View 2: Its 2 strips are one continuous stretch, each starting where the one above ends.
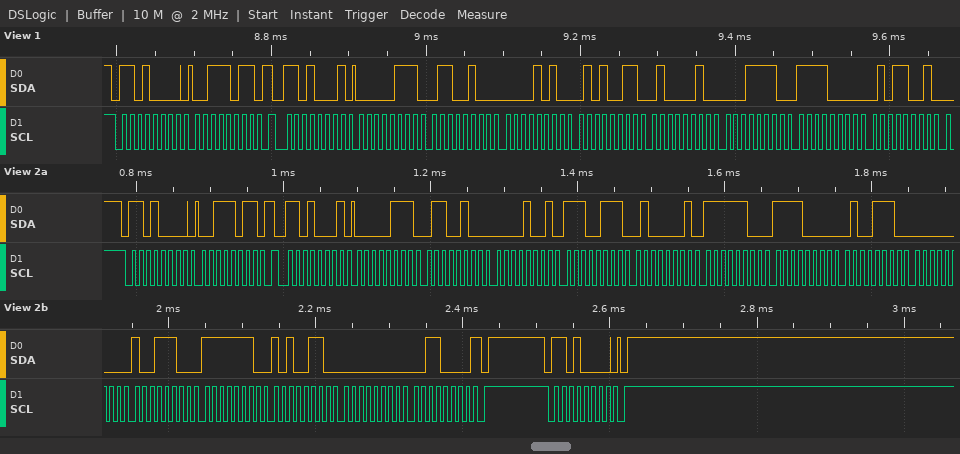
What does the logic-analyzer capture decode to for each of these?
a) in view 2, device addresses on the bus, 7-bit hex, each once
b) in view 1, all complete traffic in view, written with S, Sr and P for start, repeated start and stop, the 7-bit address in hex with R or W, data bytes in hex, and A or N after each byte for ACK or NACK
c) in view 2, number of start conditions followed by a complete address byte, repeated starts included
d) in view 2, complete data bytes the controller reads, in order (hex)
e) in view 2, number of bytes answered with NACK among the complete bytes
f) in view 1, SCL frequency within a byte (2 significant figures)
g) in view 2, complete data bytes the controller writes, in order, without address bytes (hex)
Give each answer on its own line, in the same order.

0x68
S 68W A 3B A Sr 68R A 07 A 64 A 0A A 53 A 42 A 1E A F0 A 59 A
3
07 64 09 E7 41 FC F0 4E 00 9C FE A6 00 30
1
100 kHz
3B
